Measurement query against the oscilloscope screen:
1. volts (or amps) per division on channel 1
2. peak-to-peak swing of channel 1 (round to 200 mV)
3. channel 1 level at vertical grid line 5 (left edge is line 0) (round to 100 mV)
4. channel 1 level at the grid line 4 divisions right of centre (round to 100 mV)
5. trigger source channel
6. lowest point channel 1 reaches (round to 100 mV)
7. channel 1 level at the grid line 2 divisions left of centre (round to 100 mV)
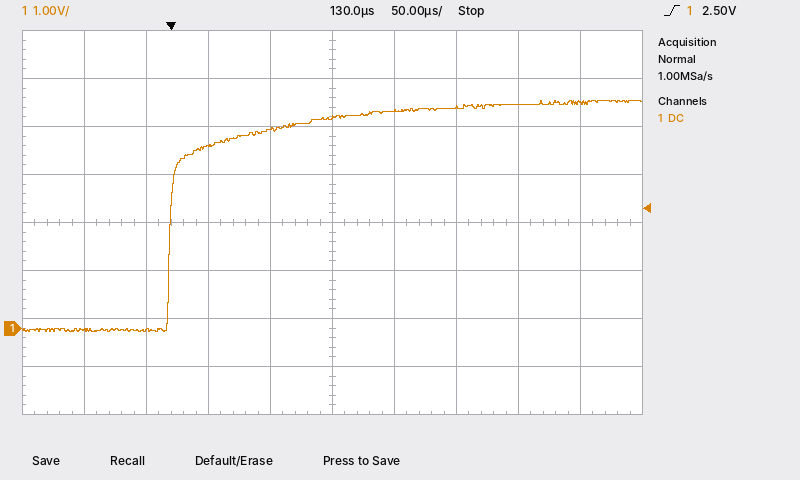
1 V
4.8 V
4.4 V
4.7 V
channel 1
-100 mV
3.8 V
